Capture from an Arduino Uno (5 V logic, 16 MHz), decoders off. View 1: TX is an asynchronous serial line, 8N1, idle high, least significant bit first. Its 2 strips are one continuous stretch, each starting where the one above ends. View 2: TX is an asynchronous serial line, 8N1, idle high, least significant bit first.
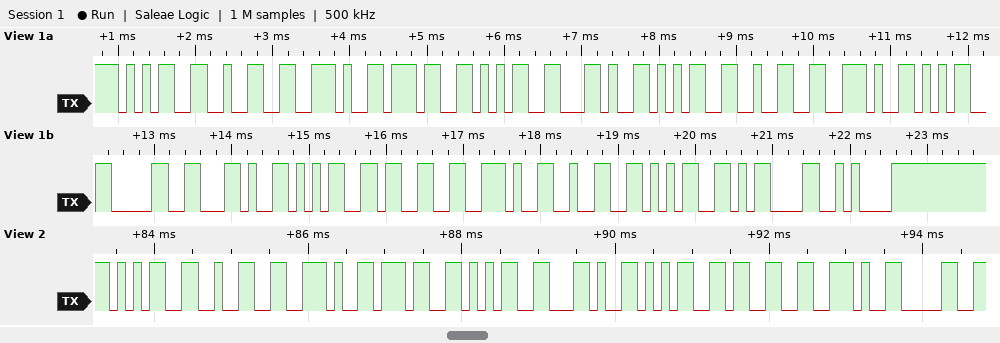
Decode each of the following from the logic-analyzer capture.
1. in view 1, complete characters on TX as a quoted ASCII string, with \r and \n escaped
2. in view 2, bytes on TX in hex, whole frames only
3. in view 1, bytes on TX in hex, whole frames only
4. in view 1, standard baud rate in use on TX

"52.75,52.50,53.25\r\n"
35 32 2E 37 35 2C 35 33 2E 30
35 32 2E 37 35 2C 35 32 2E 35 30 2C 35 33 2E 32 35 0D 0A
9600 baud
